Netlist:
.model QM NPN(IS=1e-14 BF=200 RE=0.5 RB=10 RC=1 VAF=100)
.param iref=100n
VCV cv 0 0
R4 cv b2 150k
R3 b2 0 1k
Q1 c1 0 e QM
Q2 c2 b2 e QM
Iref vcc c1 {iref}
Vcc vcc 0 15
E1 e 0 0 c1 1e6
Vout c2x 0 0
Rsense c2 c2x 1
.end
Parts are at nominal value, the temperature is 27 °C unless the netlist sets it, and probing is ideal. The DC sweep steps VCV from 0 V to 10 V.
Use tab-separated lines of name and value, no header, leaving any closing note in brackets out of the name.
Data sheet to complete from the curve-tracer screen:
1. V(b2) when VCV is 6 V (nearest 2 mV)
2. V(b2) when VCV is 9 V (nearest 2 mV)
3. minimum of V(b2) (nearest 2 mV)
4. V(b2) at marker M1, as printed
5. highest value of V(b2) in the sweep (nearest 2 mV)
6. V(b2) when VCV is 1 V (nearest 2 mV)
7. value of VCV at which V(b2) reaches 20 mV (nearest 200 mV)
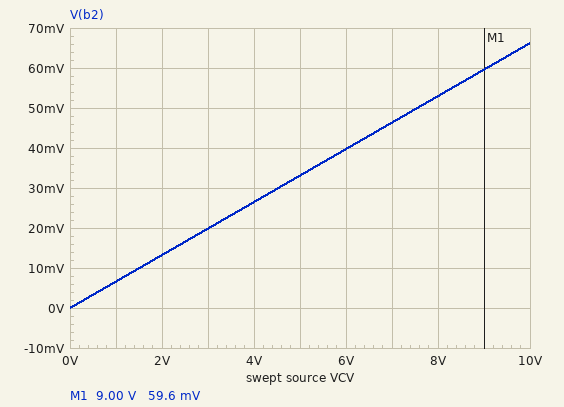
V(b2) when VCV is 6 V	40 mV
V(b2) when VCV is 9 V	60 mV
minimum of V(b2)	0 V
V(b2) at marker M1, as printed	59.6 mV
highest value of V(b2) in the sweep	66 mV
V(b2) when VCV is 1 V	6 mV
value of VCV at which V(b2) reaches 20 mV	3.0 V
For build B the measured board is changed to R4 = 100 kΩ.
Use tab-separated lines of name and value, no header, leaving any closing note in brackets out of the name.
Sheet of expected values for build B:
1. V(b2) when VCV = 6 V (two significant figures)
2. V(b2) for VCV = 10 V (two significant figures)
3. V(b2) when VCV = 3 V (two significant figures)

V(b2) when VCV = 6 V	59 mV
V(b2) for VCV = 10 V	99 mV
V(b2) when VCV = 3 V	30 mV
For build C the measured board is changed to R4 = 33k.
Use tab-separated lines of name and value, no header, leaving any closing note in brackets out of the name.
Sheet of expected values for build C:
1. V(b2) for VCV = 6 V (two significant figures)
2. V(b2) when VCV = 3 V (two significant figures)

V(b2) for VCV = 6 V	180 mV
V(b2) when VCV = 3 V	88 mV
